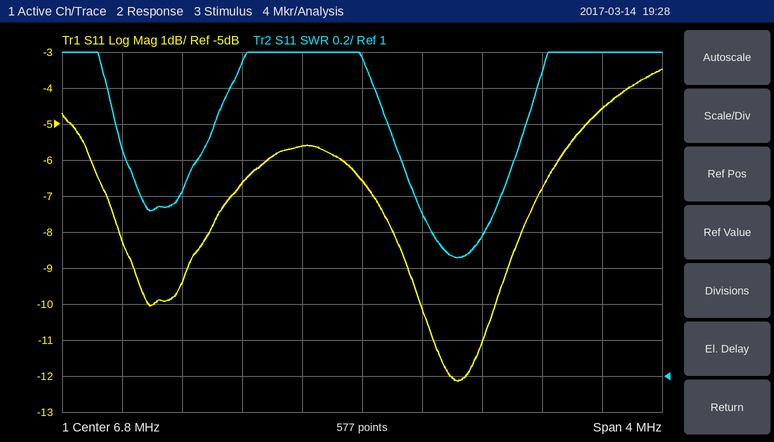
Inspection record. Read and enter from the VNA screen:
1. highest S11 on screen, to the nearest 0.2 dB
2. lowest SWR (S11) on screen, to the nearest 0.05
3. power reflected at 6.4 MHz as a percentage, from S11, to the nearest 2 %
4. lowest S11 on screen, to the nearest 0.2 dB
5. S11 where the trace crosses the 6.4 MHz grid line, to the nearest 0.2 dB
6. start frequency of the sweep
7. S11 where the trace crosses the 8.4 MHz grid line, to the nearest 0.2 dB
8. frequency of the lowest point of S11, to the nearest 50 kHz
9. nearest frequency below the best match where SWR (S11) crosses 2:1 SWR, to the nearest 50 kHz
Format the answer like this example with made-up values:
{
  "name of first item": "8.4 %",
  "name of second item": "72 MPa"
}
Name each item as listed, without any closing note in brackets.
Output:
{
  "highest S11 on screen, to the nearest 0.2 dB": "-3.4 dB",
  "lowest SWR (S11) on screen, to the nearest 0.05": "1.65",
  "power reflected at 6.4 MHz as a percentage, from S11, to the nearest 2 %": "28 %",
  "lowest S11 on screen, to the nearest 0.2 dB": "-12.2 dB",
  "S11 where the trace crosses the 6.4 MHz grid line, to the nearest 0.2 dB": "-5.6 dB",
  "start frequency of the sweep": "4.8 MHz",
  "S11 where the trace crosses the 8.4 MHz grid line, to the nearest 0.2 dB": "-4.6 dB",
  "frequency of the lowest point of S11, to the nearest 50 kHz": "7.45 MHz",
  "nearest frequency below the best match where SWR (S11) crosses 2:1 SWR, to the nearest 50 kHz": "7.15 MHz"
}
